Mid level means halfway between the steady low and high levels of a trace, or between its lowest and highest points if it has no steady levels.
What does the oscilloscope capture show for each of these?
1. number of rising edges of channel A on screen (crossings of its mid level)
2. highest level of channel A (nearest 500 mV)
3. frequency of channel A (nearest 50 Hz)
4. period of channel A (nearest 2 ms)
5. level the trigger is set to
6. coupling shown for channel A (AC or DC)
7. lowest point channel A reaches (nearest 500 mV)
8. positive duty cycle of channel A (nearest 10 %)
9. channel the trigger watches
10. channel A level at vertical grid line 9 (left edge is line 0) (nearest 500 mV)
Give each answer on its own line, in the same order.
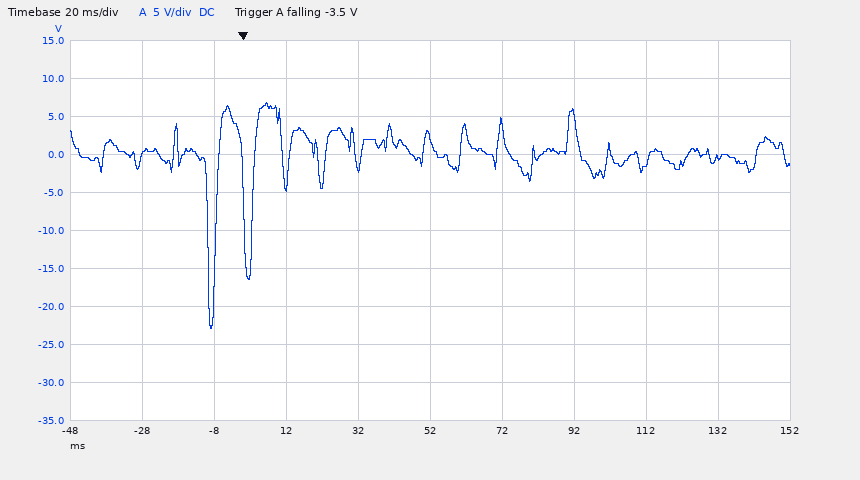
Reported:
2
7.0 V
100 Hz
10 ms
-3.5 V
DC
-23.0 V
80 %
channel A
-500 mV
